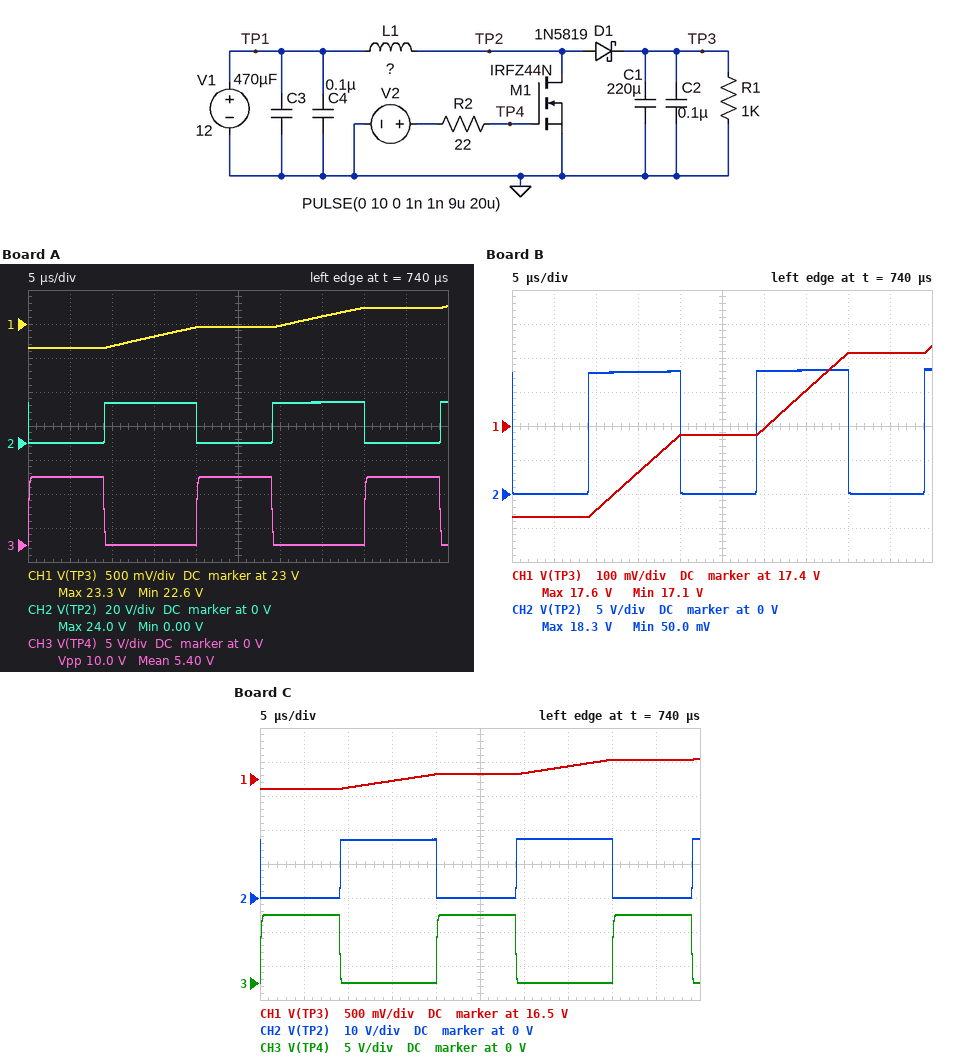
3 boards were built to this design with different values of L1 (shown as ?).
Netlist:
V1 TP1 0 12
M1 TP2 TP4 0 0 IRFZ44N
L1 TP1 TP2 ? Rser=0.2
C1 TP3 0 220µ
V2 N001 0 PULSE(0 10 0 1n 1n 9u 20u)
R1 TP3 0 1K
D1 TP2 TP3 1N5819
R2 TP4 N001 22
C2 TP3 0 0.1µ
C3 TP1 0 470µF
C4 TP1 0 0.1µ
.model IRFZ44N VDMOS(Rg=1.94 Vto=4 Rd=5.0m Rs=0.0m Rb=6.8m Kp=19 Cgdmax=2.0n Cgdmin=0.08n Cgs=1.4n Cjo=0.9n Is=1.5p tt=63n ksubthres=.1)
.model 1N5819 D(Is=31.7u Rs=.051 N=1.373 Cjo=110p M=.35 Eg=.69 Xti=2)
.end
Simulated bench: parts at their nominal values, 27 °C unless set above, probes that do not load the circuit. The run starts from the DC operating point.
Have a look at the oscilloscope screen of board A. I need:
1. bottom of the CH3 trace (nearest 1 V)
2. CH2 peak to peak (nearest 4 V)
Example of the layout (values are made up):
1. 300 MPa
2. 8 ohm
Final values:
1. 0 V
2. 24 V
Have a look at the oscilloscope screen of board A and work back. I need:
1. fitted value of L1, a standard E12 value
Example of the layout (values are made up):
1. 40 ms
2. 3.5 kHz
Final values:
1. 180 µH
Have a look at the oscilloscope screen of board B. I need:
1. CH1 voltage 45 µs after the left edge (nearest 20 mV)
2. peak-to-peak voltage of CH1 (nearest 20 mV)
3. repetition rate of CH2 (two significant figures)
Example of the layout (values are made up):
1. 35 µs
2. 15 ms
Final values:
1. 17.62 V
2. 500 mV
3. 50 kHz
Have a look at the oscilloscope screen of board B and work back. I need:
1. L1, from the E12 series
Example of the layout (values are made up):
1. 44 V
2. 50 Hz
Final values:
1. 560 µH
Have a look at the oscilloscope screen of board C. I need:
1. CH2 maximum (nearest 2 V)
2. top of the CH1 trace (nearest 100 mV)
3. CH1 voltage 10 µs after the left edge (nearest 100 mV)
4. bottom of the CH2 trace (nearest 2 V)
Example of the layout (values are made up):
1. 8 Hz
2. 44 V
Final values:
1. 18 V
2. 16.8 V
3. 16.4 V
4. 0 V
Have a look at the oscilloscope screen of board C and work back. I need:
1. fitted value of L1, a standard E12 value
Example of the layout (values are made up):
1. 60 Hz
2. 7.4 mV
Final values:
1. 680 µH
